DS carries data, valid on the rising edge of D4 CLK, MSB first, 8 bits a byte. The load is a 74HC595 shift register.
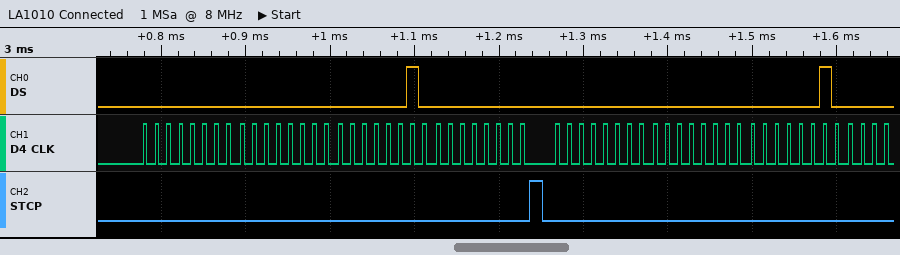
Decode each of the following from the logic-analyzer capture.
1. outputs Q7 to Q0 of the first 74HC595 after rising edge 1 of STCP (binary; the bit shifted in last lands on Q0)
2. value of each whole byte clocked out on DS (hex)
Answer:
00000000
00 00 02 00 00 00 02
